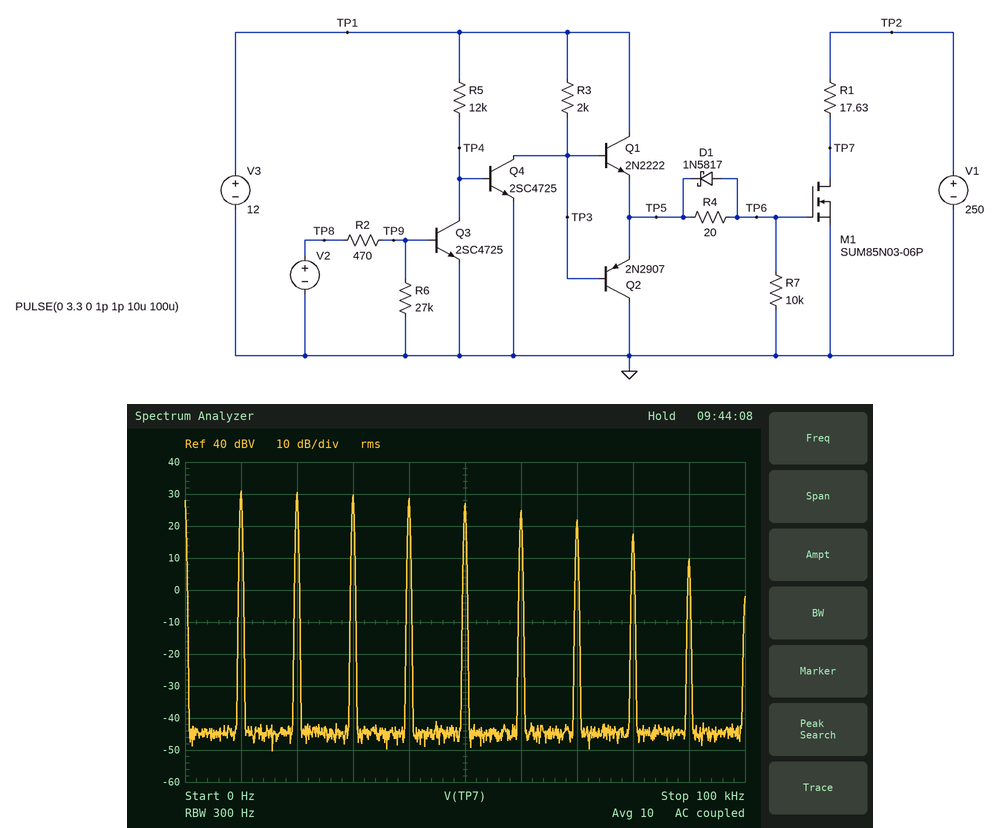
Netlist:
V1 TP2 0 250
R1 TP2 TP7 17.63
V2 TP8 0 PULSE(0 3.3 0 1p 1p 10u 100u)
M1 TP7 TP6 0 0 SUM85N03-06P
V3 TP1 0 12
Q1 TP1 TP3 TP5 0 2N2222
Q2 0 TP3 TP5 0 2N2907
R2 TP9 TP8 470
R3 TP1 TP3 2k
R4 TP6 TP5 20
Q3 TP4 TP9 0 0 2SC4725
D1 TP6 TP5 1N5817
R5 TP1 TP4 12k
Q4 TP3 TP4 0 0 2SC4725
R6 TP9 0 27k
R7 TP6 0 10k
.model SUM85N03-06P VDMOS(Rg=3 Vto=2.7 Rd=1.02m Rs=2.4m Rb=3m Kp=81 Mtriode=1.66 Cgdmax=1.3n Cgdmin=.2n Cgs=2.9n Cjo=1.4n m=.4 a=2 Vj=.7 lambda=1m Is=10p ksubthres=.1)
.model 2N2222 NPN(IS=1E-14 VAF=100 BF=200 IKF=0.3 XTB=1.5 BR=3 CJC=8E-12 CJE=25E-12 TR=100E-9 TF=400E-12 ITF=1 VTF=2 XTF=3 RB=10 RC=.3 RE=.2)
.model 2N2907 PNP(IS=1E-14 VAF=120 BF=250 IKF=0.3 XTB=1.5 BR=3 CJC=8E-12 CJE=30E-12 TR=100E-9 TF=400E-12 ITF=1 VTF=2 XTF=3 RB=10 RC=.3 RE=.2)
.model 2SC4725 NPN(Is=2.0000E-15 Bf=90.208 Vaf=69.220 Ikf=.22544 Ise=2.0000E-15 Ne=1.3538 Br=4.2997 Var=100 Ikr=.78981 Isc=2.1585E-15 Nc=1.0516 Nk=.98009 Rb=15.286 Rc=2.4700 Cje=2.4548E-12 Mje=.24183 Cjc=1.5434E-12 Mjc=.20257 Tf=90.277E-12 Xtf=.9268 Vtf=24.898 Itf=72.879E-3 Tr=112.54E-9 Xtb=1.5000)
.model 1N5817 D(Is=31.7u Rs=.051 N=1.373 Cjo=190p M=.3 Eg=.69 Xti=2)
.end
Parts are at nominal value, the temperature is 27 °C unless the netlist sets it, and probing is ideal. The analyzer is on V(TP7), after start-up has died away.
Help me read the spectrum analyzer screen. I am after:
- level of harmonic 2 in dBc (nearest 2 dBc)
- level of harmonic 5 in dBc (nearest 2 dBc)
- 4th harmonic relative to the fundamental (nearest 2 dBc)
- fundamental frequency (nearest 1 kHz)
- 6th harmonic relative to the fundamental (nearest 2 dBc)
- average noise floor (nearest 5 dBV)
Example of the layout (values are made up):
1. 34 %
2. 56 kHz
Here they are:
1. 0 dBc
2. -4 dBc
3. -2 dBc
4. 10 kHz
5. -6 dBc
6. -45 dBV
